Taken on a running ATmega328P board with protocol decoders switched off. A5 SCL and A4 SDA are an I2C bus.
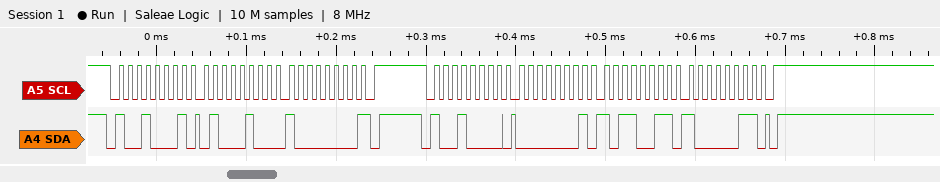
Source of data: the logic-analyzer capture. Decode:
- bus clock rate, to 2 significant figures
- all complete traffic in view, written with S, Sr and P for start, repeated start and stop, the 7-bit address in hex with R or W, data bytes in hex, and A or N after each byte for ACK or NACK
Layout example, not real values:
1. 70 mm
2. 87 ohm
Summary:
1. 100 kHz
2. S 48R A 44 A 80 N P S 48W A 01 A B3 A 83 A P
